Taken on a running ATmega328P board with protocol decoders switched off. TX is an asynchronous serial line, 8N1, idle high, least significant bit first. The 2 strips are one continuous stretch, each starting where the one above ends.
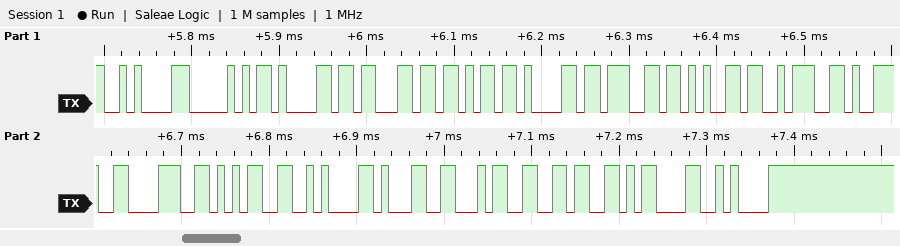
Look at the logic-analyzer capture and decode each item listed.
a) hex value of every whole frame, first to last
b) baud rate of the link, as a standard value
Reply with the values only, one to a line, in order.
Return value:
0x0A 0x50 0x61 0x63 0x6B 0x61 0x67 0x65 0x3A 0x39 0x38 0x35 0x0A 0x31 0x34 0x36 0x0D 0x0A
115200 baud
